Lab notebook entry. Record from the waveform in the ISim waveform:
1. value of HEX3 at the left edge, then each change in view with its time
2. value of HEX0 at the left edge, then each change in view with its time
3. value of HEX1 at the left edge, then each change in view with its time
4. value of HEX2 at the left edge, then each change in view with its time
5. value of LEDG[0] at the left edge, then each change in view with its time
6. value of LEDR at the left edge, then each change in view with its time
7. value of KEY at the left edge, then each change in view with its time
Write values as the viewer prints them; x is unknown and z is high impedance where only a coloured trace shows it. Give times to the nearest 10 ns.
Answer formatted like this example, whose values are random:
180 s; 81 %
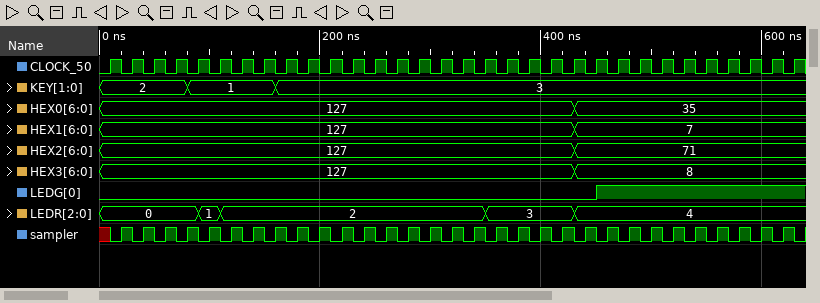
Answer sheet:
127, 8 at 430 ns; 127, 35 at 430 ns; 127, 7 at 430 ns; 127, 71 at 430 ns; 0, 1 at 450 ns; 0, 1 at 90 ns, 2 at 110 ns, 3 at 350 ns, 4 at 430 ns; 2, 1 at 80 ns, 3 at 160 ns
